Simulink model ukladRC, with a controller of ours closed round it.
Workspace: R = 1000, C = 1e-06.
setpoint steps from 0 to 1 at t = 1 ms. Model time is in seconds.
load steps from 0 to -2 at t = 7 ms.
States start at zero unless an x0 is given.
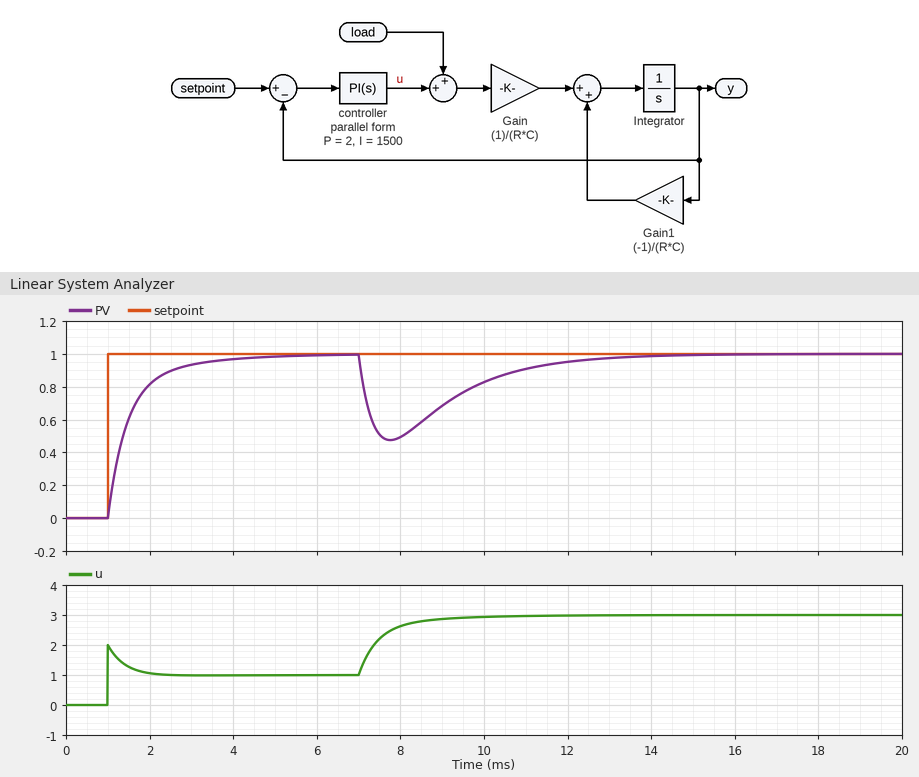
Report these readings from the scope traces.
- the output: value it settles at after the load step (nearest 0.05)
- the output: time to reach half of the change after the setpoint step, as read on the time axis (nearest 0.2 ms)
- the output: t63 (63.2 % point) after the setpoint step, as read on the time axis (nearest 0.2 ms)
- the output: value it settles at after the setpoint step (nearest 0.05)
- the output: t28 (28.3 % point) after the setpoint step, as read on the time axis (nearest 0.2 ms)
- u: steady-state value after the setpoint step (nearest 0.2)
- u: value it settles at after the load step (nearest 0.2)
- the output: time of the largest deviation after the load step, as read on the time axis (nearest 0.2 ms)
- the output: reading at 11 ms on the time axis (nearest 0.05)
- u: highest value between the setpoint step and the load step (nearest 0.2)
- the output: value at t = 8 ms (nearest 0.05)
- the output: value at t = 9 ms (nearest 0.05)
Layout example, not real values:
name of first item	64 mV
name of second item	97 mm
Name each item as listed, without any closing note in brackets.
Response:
the output: value it settles at after the load step	1.00
the output: time to reach half of the change after the setpoint step, as read on the time axis	1.4 ms
the output: t63 (63.2 % point) after the setpoint step, as read on the time axis	1.6 ms
the output: value it settles at after the setpoint step	1.00
the output: t28 (28.3 % point) after the setpoint step, as read on the time axis	1.2 ms
u: steady-state value after the setpoint step	1.0
u: value it settles at after the load step	3.0
the output: time of the largest deviation after the load step, as read on the time axis	7.8 ms
the output: reading at 11 ms on the time axis	0.90
u: highest value between the setpoint step and the load step	2.0
the output: value at t = 8 ms	0.50
the output: value at t = 9 ms	0.70
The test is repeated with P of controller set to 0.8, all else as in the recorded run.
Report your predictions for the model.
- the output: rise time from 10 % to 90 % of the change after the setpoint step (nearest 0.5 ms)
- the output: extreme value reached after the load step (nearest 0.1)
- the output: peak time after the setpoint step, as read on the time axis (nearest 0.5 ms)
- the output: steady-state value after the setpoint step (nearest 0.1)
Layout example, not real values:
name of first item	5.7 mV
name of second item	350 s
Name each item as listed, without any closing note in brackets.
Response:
the output: rise time from 10 % to 90 % of the change after the setpoint step	1.5 ms
the output: extreme value reached after the load step	0.3
the output: peak time after the setpoint step, as read on the time axis	4.0 ms
the output: steady-state value after the setpoint step	1.0
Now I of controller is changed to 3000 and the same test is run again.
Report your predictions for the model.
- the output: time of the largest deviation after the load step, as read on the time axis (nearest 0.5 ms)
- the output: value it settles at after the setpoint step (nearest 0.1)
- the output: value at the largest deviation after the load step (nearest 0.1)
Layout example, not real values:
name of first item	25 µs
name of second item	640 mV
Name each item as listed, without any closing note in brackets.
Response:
the output: time of the largest deviation after the load step, as read on the time axis	7.5 ms
the output: value it settles at after the setpoint step	1.0
the output: value at the largest deviation after the load step	0.5
